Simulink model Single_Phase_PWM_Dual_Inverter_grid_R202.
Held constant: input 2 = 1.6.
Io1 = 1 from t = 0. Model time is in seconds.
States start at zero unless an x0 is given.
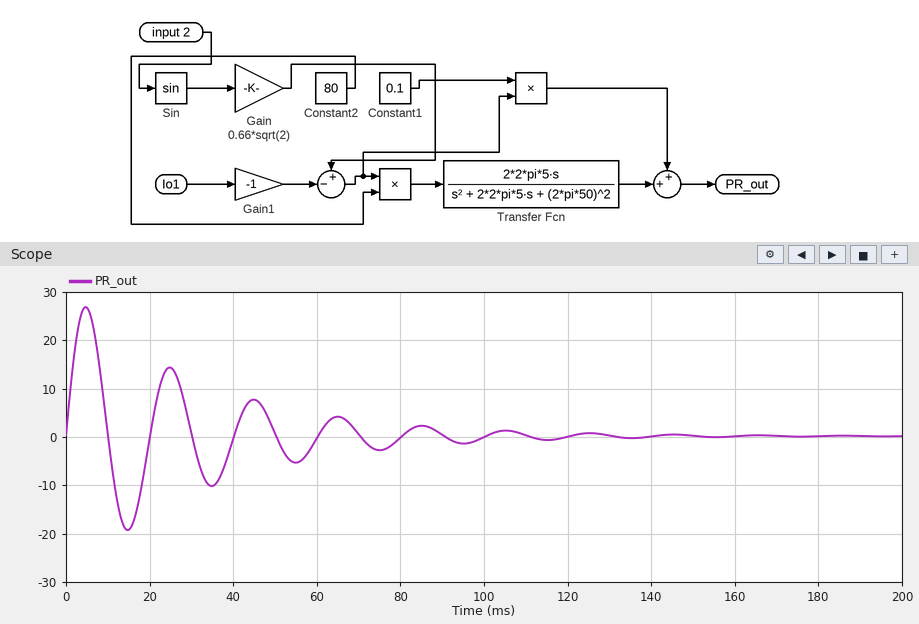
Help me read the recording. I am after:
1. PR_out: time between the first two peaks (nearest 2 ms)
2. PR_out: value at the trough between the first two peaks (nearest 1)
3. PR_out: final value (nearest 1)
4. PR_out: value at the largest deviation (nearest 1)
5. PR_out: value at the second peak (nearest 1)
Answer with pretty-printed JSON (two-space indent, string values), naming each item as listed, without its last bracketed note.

{
  "PR_out: time between the first two peaks": "20 ms",
  "PR_out: value at the trough between the first two peaks": "-19",
  "PR_out: final value": "0",
  "PR_out: value at the largest deviation": "27",
  "PR_out: value at the second peak": "14"
}
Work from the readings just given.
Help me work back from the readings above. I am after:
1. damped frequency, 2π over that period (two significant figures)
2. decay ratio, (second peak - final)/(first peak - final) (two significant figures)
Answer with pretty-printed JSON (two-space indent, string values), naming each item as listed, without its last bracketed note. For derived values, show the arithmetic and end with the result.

{
  "damped frequency, 2π over that period": "2π / 20 = 0.31 rad/ms",
  "decay ratio, (second peak - final)/(first peak - final)": "(14 - 0) / (27 - 0) = 0.52"
}
